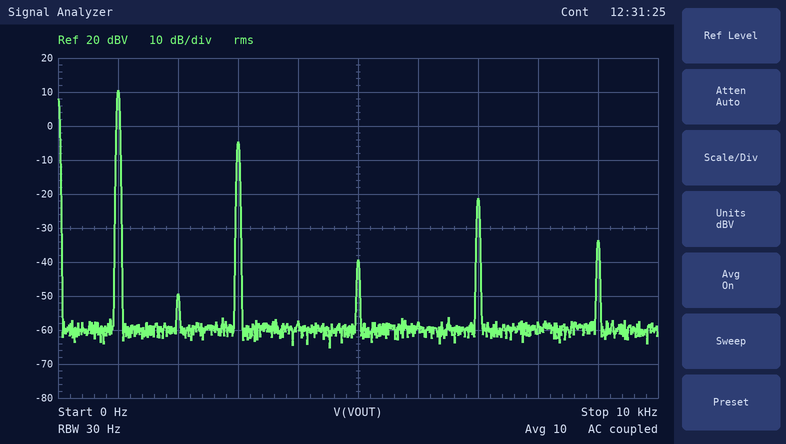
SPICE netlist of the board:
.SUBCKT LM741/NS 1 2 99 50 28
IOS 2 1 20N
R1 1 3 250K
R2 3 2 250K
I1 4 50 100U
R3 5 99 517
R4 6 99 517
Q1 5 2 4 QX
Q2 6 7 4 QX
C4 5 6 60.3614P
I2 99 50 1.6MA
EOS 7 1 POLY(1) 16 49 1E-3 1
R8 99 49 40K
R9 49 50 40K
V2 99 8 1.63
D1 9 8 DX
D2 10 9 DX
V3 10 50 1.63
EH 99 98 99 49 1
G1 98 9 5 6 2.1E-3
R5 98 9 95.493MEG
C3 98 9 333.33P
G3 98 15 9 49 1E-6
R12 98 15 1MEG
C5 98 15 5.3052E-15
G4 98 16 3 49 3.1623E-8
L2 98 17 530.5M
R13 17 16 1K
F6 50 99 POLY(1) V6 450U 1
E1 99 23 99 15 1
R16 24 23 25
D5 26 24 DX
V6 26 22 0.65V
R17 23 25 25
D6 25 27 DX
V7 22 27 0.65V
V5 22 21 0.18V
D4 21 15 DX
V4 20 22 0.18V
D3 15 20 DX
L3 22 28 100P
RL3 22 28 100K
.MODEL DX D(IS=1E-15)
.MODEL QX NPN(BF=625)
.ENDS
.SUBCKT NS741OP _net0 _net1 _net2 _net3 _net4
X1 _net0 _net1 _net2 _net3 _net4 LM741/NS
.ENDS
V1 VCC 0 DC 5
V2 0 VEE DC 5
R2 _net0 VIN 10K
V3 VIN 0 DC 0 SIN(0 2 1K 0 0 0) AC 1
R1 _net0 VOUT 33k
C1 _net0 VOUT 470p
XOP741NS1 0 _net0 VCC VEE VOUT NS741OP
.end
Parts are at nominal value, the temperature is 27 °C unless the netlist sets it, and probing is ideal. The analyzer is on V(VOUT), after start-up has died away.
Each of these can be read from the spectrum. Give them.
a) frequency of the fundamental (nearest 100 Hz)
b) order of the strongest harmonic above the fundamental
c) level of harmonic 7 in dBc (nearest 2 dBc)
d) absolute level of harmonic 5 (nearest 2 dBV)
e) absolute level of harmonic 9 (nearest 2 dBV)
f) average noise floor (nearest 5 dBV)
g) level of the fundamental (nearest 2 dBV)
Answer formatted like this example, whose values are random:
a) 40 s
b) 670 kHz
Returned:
a) 1.0 kHz
b) 3
c) -32 dBc
d) -40 dBV
e) -34 dBV
f) -60 dBV
g) 10 dBV
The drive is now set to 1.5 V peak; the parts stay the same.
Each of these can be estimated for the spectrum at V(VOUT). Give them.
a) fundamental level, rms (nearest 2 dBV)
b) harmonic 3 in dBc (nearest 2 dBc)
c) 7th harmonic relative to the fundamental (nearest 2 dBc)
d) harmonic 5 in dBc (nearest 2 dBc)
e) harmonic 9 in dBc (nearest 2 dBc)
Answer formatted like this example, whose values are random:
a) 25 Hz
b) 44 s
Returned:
a) 10 dBV
b) -22 dBc
c) -50 dBc
d) -30 dBc
e) -42 dBc
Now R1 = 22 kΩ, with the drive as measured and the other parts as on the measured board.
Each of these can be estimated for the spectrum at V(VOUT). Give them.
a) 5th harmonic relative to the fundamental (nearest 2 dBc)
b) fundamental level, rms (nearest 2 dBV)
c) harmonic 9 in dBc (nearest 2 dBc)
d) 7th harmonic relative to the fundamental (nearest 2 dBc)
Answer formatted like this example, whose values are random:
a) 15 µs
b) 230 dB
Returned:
a) -34 dBc
b) 10 dBV
c) -50 dBc
d) -40 dBc
